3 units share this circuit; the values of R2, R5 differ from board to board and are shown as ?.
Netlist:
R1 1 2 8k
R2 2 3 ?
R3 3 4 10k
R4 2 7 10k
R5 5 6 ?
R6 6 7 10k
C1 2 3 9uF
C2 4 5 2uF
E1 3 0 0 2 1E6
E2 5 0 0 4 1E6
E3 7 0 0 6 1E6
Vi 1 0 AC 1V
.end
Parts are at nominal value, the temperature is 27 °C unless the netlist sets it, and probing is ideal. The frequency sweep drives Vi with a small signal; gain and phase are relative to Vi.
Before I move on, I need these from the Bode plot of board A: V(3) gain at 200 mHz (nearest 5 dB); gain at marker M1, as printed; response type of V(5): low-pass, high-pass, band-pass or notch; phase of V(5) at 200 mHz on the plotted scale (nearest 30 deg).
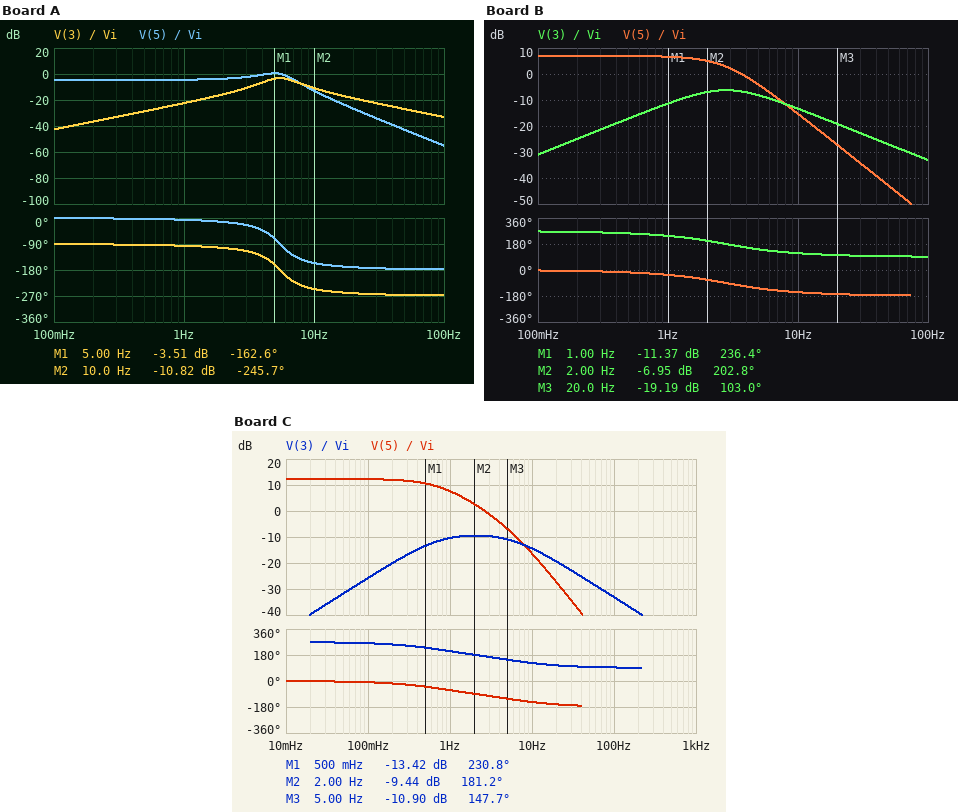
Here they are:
-35 dB
-3.51 dB
low-pass
0 deg
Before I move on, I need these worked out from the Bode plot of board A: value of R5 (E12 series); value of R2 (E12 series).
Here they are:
4.7 kΩ
5.6 kΩ
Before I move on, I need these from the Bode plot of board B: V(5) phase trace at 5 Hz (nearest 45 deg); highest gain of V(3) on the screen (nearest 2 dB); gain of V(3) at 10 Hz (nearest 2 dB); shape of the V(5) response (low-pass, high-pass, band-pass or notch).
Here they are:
-135 deg
-6 dB
-14 dB
low-pass
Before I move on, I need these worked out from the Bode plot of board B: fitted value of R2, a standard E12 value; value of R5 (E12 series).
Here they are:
3.9 kΩ
18 kΩ
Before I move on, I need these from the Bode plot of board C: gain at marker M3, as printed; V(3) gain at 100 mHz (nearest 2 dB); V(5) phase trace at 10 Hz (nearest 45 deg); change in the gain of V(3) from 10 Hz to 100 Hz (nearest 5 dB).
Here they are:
-10.90 dB
-26 dB
-135 deg
-20 dB
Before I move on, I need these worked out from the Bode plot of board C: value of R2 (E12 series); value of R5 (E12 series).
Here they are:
2.7 kΩ
33 kΩ
